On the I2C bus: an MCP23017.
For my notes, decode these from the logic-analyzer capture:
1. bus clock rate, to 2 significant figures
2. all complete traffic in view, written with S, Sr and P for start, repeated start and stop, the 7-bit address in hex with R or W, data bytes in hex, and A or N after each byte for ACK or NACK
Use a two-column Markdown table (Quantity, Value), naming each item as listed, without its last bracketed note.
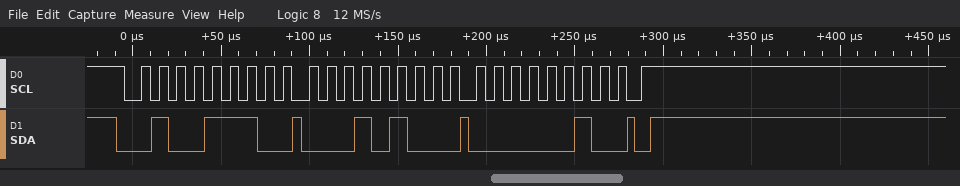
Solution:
| Quantity | Value |
|---|---|
| bus clock rate, to 2 significant figures | 100 kHz |
| all complete traffic in view, written with S, Sr and P for start, repeated start and stop, the 7-bit address in hex with R or W, data bytes in hex, and A or N after each byte for ACK or NACK | S 27W A 14 A 02 A P |
